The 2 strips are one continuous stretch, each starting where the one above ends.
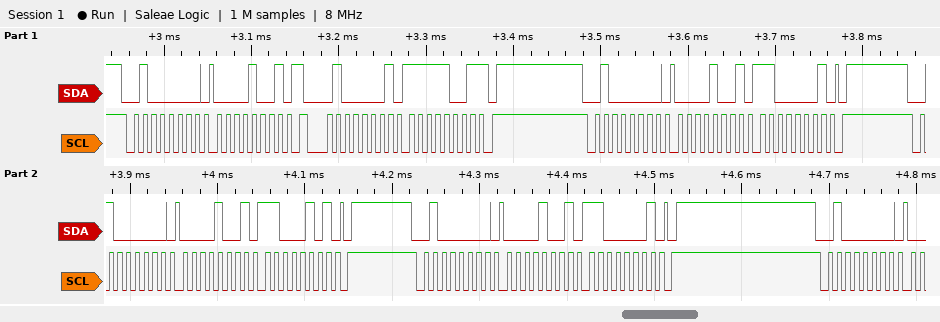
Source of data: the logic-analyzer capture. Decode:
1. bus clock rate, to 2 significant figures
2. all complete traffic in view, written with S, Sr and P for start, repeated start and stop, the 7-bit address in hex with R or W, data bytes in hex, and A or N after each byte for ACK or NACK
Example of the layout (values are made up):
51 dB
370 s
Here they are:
100 kHz
S 20W A 09 A Sr 20R A F9 N P S 20W A 09 A C1 A P S 20W A 09 A C5 A P S 20W A 09 A C1 A P S 20W A
